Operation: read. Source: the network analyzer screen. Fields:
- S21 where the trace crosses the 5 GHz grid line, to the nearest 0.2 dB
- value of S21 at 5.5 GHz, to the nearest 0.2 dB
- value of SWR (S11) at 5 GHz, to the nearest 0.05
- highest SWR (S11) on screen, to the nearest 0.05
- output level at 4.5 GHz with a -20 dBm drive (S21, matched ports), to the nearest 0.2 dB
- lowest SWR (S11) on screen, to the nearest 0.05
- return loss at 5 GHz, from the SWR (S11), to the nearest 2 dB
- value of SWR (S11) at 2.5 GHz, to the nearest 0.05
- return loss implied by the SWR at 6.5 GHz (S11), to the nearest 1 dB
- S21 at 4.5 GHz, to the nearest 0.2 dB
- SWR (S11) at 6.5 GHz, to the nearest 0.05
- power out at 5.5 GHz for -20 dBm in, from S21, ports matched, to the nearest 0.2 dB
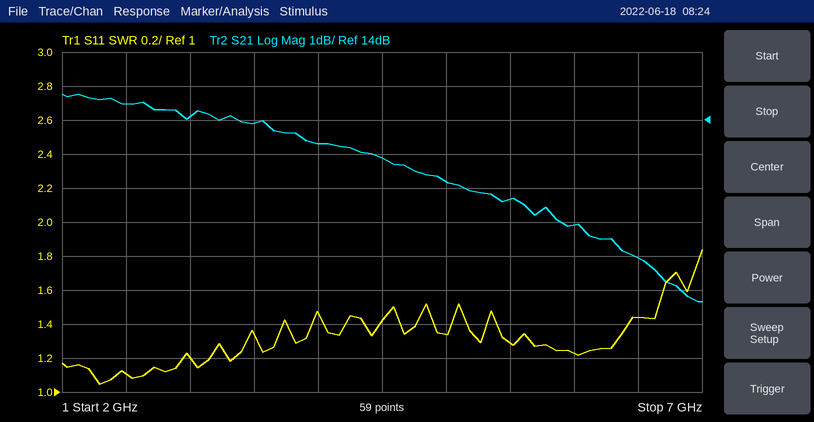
12.2 dB
11.6 dB
1.35
1.85
-7.2 dBm
1.05
16 dB
1.10
15 dB
12.8 dB
1.45
-8.4 dBm
